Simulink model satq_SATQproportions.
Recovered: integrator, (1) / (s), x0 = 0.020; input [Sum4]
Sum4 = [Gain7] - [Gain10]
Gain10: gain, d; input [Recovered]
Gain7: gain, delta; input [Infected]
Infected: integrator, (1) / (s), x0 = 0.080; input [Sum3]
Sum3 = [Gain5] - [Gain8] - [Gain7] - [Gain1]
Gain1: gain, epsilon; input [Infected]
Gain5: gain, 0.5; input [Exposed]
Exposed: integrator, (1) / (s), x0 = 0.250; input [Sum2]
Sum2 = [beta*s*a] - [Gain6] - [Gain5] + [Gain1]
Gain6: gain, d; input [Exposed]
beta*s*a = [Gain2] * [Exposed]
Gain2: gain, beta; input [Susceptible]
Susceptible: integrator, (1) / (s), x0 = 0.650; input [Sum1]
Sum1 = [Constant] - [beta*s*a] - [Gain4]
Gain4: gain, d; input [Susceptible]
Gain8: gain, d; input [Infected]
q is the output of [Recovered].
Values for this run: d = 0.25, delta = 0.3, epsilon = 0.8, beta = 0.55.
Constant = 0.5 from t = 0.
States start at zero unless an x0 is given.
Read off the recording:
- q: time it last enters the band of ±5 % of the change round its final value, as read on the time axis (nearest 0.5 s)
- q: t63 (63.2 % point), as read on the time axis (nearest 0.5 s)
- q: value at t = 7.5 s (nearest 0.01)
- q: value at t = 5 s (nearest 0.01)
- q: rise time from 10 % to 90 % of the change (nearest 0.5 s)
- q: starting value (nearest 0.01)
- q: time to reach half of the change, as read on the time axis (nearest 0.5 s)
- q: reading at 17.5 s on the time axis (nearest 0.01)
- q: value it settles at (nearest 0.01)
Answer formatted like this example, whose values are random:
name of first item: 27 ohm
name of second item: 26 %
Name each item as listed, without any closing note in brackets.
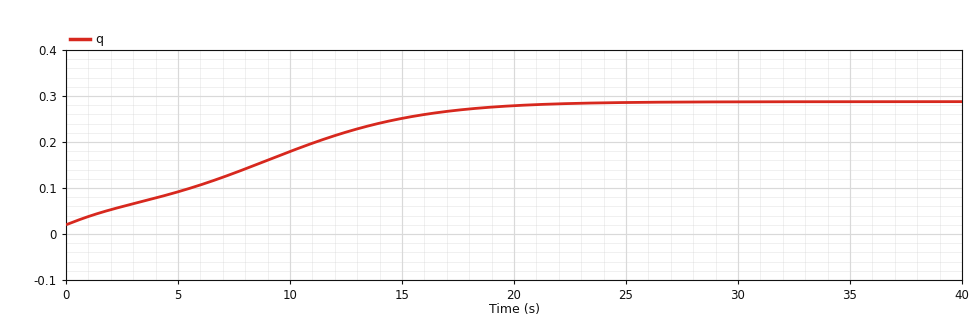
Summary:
q: time it last enters the band of ±5 % of the change round its final value, as read on the time axis: 18.5 s
q: t63 (63.2 % point), as read on the time axis: 10.5 s
q: value at t = 7.5 s: 0.13
q: value at t = 5 s: 0.09
q: rise time from 10 % to 90 % of the change: 14.5 s
q: starting value: 0.02
q: time to reach half of the change, as read on the time axis: 8.5 s
q: reading at 17.5 s on the time axis: 0.27
q: value it settles at: 0.29
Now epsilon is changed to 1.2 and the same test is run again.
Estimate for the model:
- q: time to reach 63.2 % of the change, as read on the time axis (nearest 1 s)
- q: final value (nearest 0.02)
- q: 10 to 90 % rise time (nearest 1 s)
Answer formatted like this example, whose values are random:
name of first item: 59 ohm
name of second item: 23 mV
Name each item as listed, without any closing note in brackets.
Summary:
q: time to reach 63.2 % of the change, as read on the time axis: 10 s
q: final value: 0.26
q: 10 to 90 % rise time: 14 s
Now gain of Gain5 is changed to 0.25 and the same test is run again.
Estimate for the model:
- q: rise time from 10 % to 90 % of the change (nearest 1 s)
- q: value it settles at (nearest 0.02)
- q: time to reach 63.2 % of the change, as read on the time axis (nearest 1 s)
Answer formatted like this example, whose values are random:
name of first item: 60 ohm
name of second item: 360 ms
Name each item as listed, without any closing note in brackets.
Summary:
q: rise time from 10 % to 90 % of the change: 14 s
q: value it settles at: 0.22
q: time to reach 63.2 % of the change, as read on the time axis: 10 s
